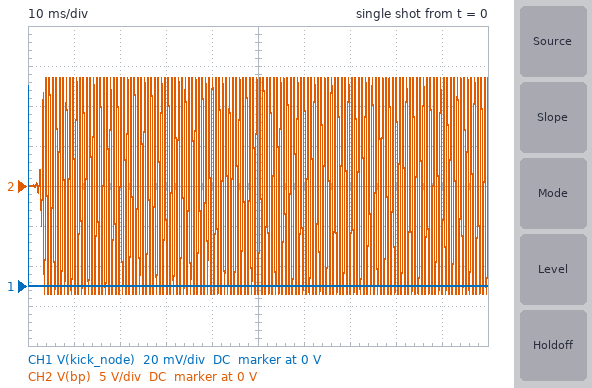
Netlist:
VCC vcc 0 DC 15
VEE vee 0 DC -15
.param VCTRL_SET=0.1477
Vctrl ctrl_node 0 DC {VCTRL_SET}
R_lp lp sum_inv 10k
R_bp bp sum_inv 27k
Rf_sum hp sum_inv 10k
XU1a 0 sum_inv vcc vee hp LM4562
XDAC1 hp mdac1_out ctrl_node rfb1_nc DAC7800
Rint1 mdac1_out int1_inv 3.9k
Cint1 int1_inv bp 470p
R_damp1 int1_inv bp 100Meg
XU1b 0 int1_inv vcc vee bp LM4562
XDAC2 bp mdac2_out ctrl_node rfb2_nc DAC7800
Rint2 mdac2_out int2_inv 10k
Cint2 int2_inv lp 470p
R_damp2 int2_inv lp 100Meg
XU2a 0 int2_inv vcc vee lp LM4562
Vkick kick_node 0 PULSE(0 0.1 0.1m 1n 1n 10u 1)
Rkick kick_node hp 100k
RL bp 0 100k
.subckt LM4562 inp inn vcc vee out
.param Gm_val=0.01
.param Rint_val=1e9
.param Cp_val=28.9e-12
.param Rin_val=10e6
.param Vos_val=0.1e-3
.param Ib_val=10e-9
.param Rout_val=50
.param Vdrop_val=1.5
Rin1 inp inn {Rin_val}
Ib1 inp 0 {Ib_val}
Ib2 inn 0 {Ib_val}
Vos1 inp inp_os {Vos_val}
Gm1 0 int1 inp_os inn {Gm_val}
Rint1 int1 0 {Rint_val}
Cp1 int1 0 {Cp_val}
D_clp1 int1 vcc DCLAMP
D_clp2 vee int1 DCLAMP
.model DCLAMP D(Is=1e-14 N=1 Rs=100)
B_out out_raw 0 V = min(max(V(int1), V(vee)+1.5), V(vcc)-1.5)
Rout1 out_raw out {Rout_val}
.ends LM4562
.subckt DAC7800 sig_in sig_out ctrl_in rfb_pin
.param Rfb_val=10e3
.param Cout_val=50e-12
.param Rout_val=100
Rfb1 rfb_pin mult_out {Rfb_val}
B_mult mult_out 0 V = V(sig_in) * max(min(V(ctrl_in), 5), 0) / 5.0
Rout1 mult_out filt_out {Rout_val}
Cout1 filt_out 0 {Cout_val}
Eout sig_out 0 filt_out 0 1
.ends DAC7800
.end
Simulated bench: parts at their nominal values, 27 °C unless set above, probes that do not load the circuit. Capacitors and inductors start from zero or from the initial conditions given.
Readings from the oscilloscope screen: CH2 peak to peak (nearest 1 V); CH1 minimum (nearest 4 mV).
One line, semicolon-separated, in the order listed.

27 V; 0 V
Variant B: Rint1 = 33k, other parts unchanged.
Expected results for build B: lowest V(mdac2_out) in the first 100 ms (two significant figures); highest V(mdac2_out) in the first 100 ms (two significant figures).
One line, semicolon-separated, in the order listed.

-260 mV; 260 mV
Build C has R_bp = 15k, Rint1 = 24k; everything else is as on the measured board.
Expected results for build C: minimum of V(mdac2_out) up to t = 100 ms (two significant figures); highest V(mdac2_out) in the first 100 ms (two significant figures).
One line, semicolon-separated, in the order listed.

-370 mV; 370 mV
